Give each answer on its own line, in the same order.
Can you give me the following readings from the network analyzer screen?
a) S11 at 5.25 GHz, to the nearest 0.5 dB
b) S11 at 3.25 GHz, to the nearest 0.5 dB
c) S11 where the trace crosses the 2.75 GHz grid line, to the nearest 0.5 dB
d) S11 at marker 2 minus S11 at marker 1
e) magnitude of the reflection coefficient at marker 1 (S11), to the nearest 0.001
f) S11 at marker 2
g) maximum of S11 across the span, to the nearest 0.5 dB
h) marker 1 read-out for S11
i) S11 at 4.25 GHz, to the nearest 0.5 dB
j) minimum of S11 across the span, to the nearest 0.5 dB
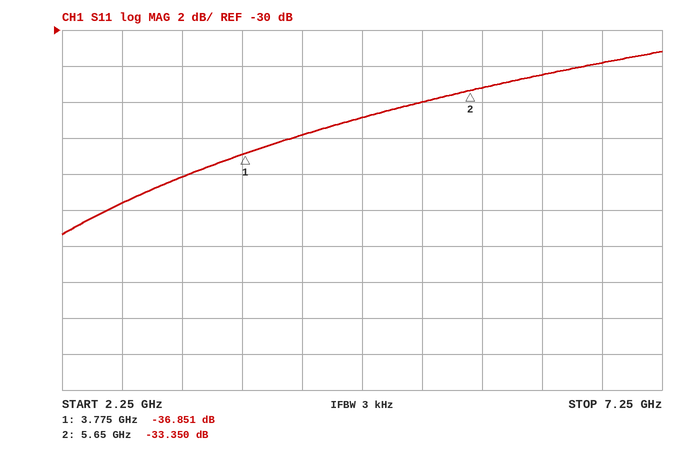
-34.0 dB
-38.0 dB
-39.5 dB
3.501 dB
0.014
-33.350 dB
-31.0 dB
-36.851 dB
-36.0 dB
-41.5 dB
